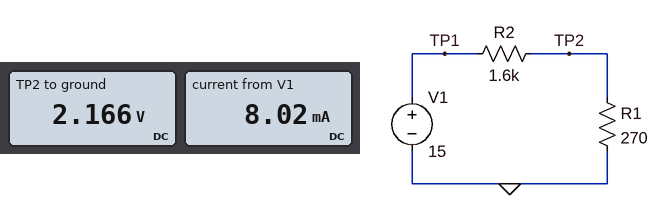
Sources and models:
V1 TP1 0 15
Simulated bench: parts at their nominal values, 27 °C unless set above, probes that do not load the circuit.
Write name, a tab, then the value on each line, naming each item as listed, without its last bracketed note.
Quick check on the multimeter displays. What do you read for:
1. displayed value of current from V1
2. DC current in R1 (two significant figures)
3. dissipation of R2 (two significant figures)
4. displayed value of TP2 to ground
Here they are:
displayed value of current from V1	8.02 mA
DC current in R1	8.0 mA
dissipation of R2	100 mW
displayed value of TP2 to ground	2.166 V
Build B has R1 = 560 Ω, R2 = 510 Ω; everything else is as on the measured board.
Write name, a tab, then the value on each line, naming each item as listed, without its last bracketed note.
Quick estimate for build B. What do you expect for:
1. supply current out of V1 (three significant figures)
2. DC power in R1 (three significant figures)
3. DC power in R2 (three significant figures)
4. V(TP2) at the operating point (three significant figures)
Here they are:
supply current out of V1	14.0 mA
DC power in R1	110 mW
DC power in R2	100 mW
V(TP2) at the operating point	7.85 V
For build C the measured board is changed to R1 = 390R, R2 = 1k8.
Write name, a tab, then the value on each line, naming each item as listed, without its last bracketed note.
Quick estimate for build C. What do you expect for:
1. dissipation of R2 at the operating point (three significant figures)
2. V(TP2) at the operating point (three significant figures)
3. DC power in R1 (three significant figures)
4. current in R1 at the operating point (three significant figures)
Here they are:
dissipation of R2 at the operating point	84.4 mW
V(TP2) at the operating point	2.67 V
DC power in R1	18.3 mW
current in R1 at the operating point	6.85 mA
